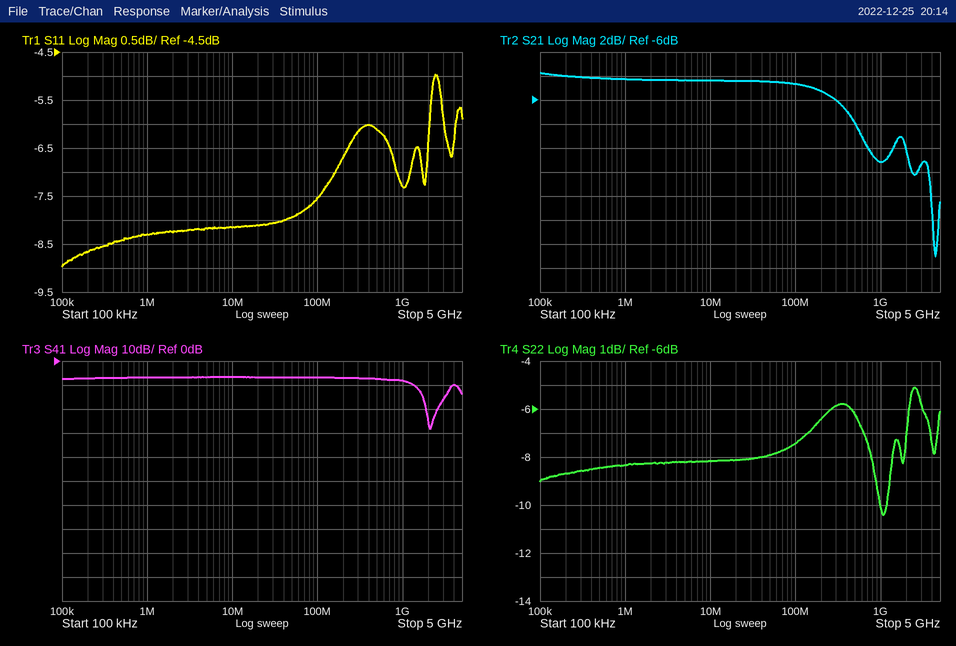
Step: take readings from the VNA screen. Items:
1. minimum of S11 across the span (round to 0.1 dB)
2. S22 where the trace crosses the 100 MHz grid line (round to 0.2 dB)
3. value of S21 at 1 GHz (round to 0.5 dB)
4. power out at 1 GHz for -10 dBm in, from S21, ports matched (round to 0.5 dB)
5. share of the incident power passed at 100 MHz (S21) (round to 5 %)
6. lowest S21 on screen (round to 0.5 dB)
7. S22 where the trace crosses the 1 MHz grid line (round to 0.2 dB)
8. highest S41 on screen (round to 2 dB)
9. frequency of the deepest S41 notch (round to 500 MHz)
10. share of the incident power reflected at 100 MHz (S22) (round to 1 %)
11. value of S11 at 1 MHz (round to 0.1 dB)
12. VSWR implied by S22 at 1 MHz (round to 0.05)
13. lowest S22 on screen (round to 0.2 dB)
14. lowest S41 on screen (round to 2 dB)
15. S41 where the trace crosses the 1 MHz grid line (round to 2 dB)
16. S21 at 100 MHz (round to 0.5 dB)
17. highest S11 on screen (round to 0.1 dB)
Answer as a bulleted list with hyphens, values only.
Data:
- -9.0 dB
- -7.4 dB
- -11.0 dB
- -21.0 dBm
- 35 %
- -19.0 dB
- -8.4 dB
- -6 dB
- 2.0 GHz
- 18 %
- -8.3 dB
- 2.25
- -10.4 dB
- -28 dB
- -6 dB
- -4.5 dB
- -5.0 dB
